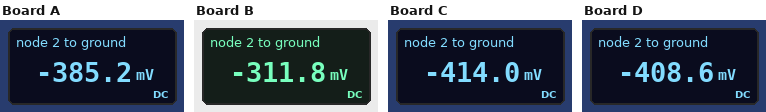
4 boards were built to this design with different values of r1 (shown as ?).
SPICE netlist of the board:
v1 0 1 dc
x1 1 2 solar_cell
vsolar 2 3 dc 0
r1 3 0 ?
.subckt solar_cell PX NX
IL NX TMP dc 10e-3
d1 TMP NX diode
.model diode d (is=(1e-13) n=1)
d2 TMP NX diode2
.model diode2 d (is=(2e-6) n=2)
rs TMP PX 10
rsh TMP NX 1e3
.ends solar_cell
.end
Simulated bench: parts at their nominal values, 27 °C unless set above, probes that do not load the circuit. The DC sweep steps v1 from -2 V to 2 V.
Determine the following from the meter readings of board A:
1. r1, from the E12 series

120 Ω
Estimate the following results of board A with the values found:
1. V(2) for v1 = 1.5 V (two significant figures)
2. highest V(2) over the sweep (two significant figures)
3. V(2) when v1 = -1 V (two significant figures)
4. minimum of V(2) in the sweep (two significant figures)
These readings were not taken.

-1.2 V
1.4 V
500 mV
-1.3 V
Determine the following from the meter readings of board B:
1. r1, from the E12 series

47 Ω
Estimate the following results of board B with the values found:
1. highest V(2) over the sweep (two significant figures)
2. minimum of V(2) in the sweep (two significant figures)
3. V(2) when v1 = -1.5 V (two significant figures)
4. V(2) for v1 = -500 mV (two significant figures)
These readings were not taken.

1.2 V
-530 mV
830 mV
47 mV
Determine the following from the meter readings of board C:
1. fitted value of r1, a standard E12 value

270 Ω
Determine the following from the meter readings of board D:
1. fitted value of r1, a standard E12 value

220 Ω
